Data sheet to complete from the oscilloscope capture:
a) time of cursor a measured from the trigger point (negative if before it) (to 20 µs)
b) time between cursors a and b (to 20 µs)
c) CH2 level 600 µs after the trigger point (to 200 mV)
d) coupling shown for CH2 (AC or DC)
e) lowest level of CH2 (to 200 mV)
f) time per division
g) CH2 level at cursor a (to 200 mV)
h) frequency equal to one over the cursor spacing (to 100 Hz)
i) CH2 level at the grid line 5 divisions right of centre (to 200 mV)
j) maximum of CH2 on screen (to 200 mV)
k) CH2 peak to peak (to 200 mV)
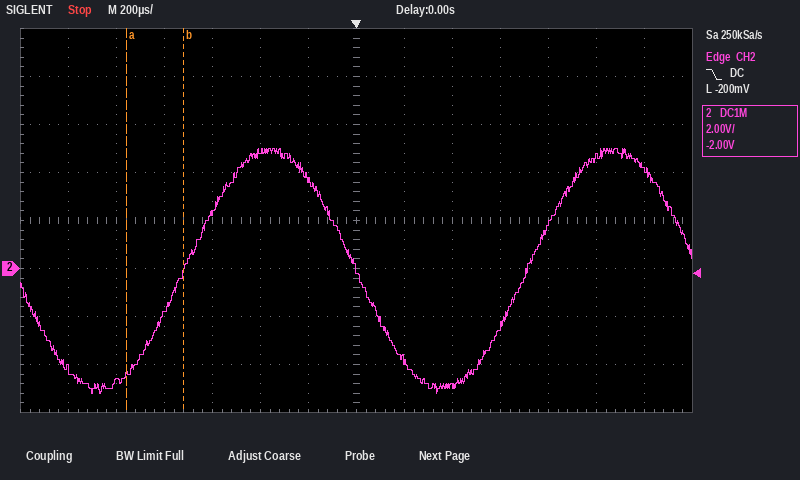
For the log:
-960 µs
240 µs
-2.4 V
DC
-5.2 V
200 µs
-4.4 V
4.2 kHz
4.6 V
5.0 V
10.2 V
